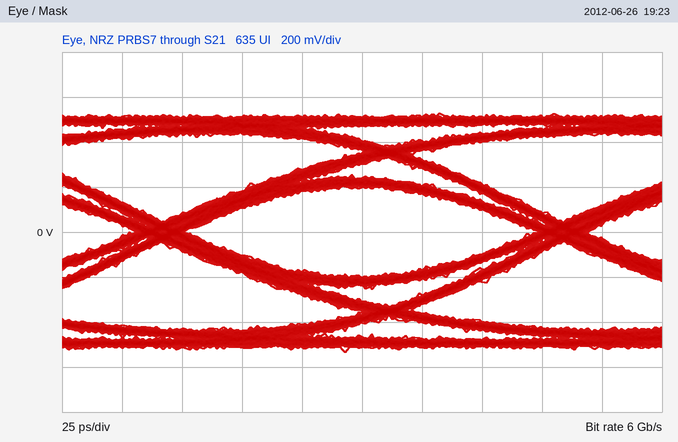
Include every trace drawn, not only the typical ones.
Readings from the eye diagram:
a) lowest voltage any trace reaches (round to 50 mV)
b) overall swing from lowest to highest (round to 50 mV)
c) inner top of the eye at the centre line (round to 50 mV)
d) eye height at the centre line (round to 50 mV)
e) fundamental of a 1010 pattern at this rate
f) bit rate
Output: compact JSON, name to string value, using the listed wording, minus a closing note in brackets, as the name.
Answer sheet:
{"lowest voltage any trace reaches": "-550 mV", "overall swing from lowest to highest": "1.05 V", "inner top of the eye at the centre line": "200 mV", "eye height at the centre line": "400 mV", "fundamental of a 1010 pattern at this rate": "3 GHz", "bit rate": "6 Gb/s"}
